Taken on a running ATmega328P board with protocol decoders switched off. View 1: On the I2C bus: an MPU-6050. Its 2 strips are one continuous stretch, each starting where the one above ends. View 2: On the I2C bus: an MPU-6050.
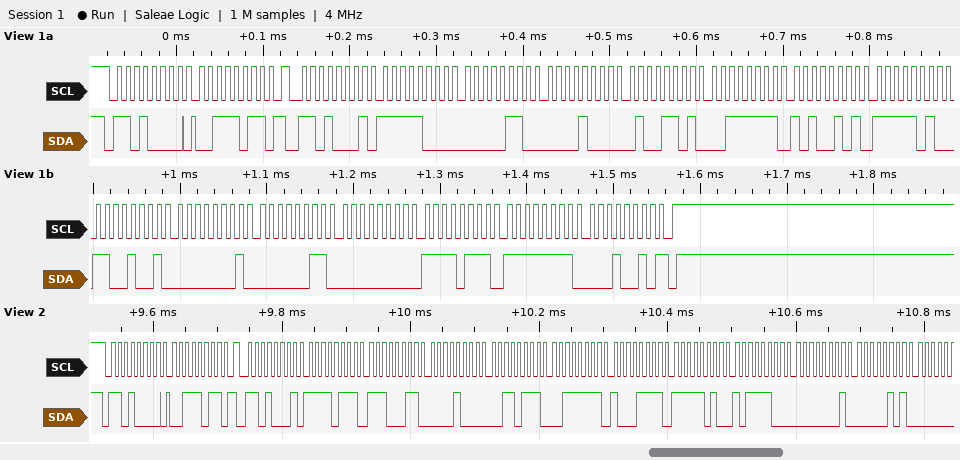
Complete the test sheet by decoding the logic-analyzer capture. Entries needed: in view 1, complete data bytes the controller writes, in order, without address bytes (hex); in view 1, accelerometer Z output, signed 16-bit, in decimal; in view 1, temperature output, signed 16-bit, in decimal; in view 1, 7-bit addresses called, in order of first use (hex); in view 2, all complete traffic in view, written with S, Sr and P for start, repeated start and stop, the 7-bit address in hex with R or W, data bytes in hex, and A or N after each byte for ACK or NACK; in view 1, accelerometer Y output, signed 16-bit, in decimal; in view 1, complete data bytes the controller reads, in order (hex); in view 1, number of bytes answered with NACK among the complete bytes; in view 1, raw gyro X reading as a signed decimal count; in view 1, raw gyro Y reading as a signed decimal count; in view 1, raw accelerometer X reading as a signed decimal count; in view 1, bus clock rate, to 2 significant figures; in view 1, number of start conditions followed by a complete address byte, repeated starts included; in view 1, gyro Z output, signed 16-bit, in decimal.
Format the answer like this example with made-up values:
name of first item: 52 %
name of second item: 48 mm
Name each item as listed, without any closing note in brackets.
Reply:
in view 1, complete data bytes the controller writes, in order, without address bytes: 3B
in view 1, accelerometer Z output, signed 16-bit, in decimal: 16293
in view 1, temperature output, signed 16-bit, in decimal: -1335
in view 1, 7-bit addresses called, in order of first use: 0x68
in view 2, all complete traffic in view, written with S, Sr and P for start, repeated start and stop, the 7-bit address in hex with R or W, data bytes in hex, and A or N after each byte for ACK or NACK: S 68W A 3B A Sr 68R A F7 A E3 A 08 A 37 A 3F A 8F A FA A BC A 01 A 05 A
in view 1, accelerometer Y output, signed 16-bit, in decimal: 2125
in view 1, complete data bytes the controller reads, in order: F8 06 08 4D 3F A5 FA C9 01 03 00 F7 FF 12
in view 1, number of bytes answered with NACK among the complete bytes: 1
in view 1, raw gyro X reading as a signed decimal count: 259
in view 1, raw gyro Y reading as a signed decimal count: 247
in view 1, raw accelerometer X reading as a signed decimal count: -2042
in view 1, bus clock rate, to 2 significant figures: 100 kHz
in view 1, number of start conditions followed by a complete address byte, repeated starts included: 2
in view 1, gyro Z output, signed 16-bit, in decimal: -238
